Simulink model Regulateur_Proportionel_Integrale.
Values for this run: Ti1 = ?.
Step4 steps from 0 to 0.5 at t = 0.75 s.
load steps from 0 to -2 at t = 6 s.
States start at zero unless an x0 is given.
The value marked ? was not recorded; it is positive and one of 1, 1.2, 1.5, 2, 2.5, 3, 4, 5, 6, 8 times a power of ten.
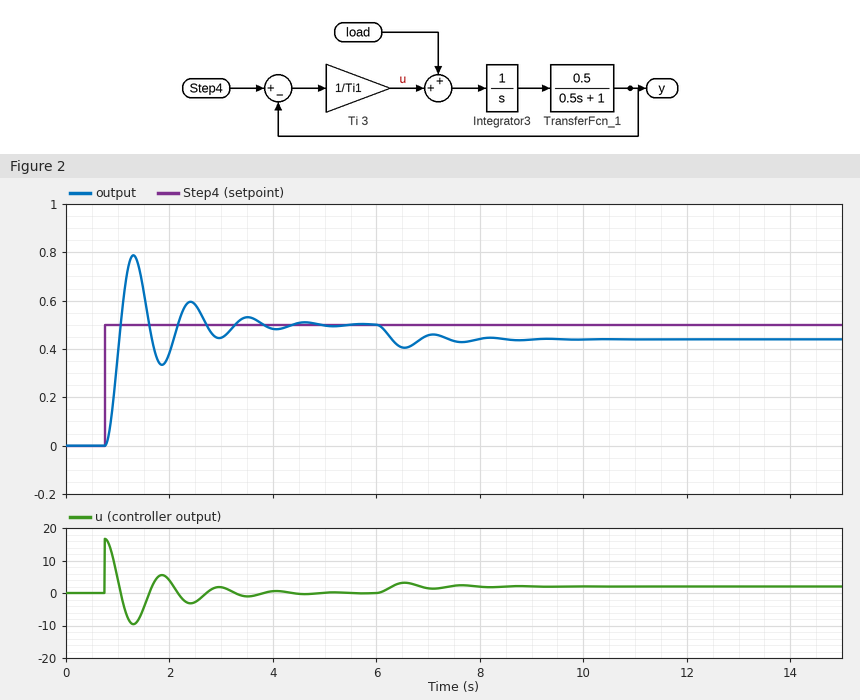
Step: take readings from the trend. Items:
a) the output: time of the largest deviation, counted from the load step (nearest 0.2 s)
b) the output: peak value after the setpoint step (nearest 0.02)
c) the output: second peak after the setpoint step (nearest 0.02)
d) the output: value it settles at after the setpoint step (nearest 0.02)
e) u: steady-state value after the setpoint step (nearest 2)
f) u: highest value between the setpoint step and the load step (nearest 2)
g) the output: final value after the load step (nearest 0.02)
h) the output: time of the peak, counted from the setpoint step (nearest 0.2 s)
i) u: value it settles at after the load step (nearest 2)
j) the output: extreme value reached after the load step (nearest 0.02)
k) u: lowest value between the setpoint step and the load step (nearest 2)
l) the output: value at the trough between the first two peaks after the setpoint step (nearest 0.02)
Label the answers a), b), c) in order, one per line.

a) 0.6 s
b) 0.78
c) 0.60
d) 0.50
e) 0
f) 16
g) 0.44
h) 0.6 s
i) 2
j) 0.40
k) -10
l) 0.34
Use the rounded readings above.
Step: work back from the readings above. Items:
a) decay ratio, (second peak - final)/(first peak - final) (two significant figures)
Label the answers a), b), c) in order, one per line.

a) 0.36
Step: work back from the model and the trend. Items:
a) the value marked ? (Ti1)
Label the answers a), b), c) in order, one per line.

a) 0.03
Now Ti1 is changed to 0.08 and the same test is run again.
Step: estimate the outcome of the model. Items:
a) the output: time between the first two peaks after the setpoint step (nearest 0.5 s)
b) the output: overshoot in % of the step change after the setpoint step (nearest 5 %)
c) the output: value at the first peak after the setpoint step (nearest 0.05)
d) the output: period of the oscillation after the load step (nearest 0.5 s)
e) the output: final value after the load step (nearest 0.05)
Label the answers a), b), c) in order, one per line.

a) 2.0 s
b) 40 %
c) 0.70
d) 2.0 s
e) 0.35
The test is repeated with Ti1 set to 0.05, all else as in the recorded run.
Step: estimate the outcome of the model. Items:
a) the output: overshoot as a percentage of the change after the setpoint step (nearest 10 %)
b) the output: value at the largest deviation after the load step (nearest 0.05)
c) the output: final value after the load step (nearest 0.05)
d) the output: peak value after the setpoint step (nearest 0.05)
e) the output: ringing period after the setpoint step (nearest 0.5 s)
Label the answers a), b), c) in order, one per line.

a) 50 %
b) 0.35
c) 0.40
d) 0.75
e) 1.5 s
